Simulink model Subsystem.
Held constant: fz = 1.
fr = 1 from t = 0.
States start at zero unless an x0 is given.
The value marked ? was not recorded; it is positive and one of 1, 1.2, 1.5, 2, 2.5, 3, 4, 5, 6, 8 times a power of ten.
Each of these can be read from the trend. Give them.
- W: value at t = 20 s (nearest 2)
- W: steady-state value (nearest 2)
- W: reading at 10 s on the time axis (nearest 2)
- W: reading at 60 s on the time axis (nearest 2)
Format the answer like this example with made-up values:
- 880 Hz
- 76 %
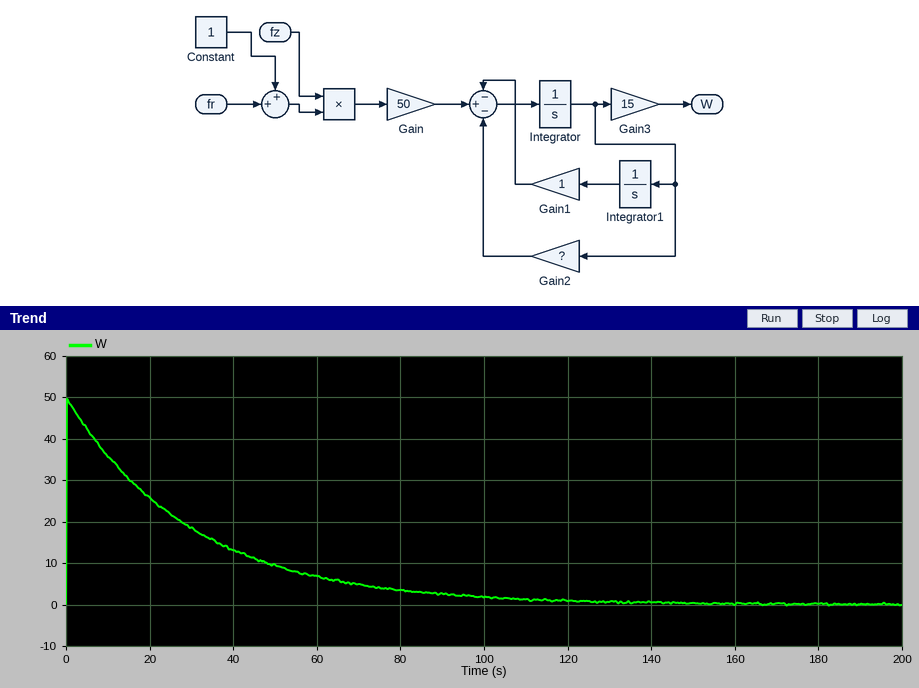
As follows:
- 26
- 0
- 36
- 6
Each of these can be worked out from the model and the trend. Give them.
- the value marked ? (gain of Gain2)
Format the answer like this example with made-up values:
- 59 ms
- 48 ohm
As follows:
- 30
